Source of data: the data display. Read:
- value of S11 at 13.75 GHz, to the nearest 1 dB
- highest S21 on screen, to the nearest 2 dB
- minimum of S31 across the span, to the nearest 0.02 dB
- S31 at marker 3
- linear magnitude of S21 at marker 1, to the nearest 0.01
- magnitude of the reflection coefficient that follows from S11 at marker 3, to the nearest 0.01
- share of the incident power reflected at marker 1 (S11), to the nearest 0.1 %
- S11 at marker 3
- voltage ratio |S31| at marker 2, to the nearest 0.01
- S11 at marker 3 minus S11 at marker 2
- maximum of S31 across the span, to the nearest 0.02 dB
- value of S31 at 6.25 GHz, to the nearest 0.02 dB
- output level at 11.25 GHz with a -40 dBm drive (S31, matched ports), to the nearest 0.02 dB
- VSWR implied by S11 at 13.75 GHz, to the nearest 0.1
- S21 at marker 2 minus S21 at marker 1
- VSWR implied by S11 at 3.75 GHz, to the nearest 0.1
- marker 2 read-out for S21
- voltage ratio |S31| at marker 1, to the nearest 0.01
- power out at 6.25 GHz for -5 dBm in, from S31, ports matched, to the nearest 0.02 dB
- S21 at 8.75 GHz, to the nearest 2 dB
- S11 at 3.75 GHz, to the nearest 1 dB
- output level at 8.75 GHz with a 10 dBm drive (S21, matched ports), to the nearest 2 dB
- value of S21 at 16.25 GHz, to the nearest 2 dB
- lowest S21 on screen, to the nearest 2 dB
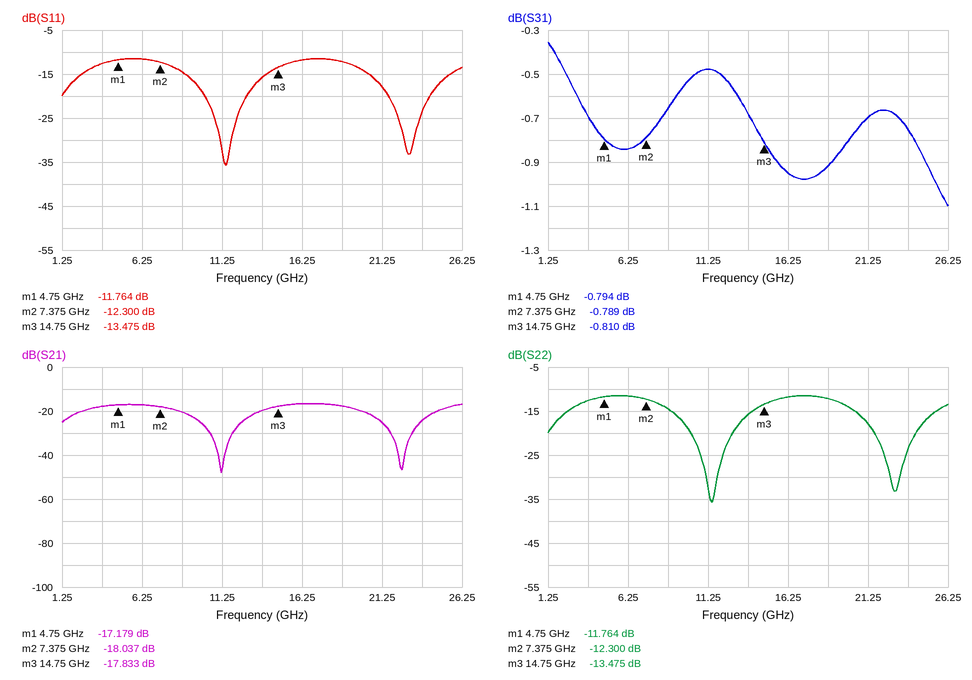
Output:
-16 dB
-16 dB
-1.10 dB
-0.810 dB
0.14
0.21
6.7 %
-13.475 dB
0.91
-1.175 dB
-0.36 dB
-0.84 dB
-40.48 dBm
1.4
-0.858 dB
1.6
-18.037 dB
0.91
-5.84 dBm
-20 dB
-13 dB
-10 dBm
-16 dB
-48 dB
